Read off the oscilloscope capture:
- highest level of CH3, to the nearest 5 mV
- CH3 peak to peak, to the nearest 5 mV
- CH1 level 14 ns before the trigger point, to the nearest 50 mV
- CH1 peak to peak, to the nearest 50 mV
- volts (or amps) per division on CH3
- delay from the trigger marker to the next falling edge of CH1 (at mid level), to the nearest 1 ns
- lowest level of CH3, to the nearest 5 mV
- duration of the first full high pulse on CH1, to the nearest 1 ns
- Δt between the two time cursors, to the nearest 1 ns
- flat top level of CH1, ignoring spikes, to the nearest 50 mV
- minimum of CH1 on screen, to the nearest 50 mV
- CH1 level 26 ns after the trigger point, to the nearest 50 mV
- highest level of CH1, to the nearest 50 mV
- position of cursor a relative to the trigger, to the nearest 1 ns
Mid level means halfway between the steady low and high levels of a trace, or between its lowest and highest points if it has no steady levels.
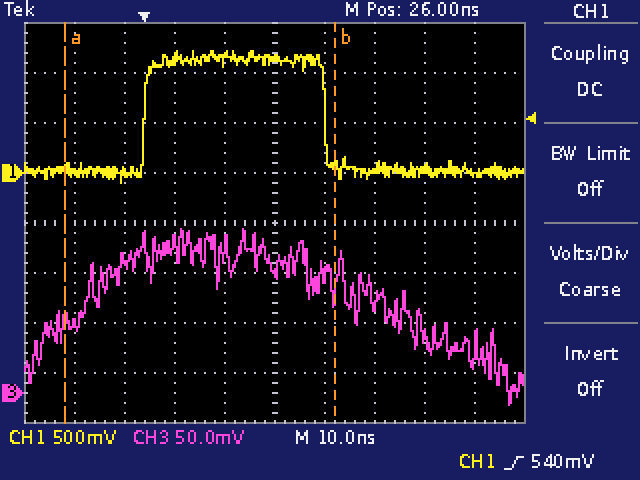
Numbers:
165 mV
175 mV
0 mV
1.30 V
50 mV
36 ns
-10 mV
36 ns
54 ns
1.15 V
-100 mV
1.15 V
1.20 V
-16 ns
